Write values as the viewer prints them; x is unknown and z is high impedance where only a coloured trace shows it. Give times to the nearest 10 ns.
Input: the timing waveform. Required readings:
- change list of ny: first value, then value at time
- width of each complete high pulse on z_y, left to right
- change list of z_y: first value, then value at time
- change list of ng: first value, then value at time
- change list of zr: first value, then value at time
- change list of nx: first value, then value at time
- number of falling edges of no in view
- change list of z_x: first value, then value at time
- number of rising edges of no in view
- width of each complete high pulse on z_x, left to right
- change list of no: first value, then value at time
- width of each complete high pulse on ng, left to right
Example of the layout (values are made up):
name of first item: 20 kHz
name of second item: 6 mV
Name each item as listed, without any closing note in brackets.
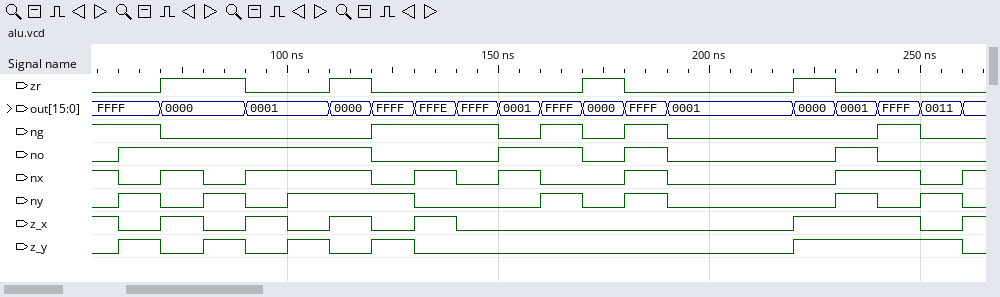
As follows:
change list of ny: first value, then value at time: 0, 1 at 60 ns, 0 at 70 ns, 1 at 80 ns, 0 at 90 ns, 1 at 100 ns, 0 at 130 ns, 1 at 160 ns, 0 at 170 ns, 1 at 180 ns, 0 at 190 ns, 1 at 230 ns, 0 at 240 ns, 1 at 250 ns, 0 at 260 ns
width of each complete high pulse on z_y, left to right: 10 ns, 10 ns, 10 ns, 10 ns, 40 ns
change list of z_y: first value, then value at time: 0, 1 at 60 ns, 0 at 70 ns, 1 at 80 ns, 0 at 90 ns, 1 at 100 ns, 0 at 110 ns, 1 at 120 ns, 0 at 130 ns, 1 at 220 ns, 0 at 260 ns
change list of ng: first value, then value at time: 1, 0 at 70 ns, 1 at 120 ns, 0 at 150 ns, 1 at 160 ns, 0 at 170 ns, 1 at 180 ns, 0 at 190 ns, 1 at 240 ns, 0 at 250 ns
change list of zr: first value, then value at time: 0, 1 at 70 ns, 0 at 90 ns, 1 at 110 ns, 0 at 120 ns, 1 at 170 ns, 0 at 180 ns, 1 at 220 ns, 0 at 230 ns
change list of nx: first value, then value at time: 1, 0 at 60 ns, 1 at 70 ns, 0 at 80 ns, 1 at 90 ns, 0 at 120 ns, 1 at 130 ns, 0 at 140 ns, 1 at 150 ns, 0 at 160 ns, 1 at 180 ns, 0 at 190 ns, 1 at 230 ns, 0 at 250 ns, 1 at 260 ns
number of falling edges of no in view: 4
change list of z_x: first value, then value at time: 1, 0 at 60 ns, 1 at 70 ns, 0 at 80 ns, 1 at 90 ns, 0 at 100 ns, 1 at 110 ns, 0 at 120 ns, 1 at 130 ns, 0 at 140 ns, 1 at 220 ns, 0 at 250 ns, 1 at 260 ns
number of rising edges of no in view: 4
width of each complete high pulse on z_x, left to right: 10 ns, 10 ns, 10 ns, 10 ns, 30 ns
change list of no: first value, then value at time: 0, 1 at 60 ns, 0 at 120 ns, 1 at 150 ns, 0 at 170 ns, 1 at 180 ns, 0 at 190 ns, 1 at 230 ns, 0 at 240 ns
width of each complete high pulse on ng, left to right: 30 ns, 10 ns, 10 ns, 10 ns
